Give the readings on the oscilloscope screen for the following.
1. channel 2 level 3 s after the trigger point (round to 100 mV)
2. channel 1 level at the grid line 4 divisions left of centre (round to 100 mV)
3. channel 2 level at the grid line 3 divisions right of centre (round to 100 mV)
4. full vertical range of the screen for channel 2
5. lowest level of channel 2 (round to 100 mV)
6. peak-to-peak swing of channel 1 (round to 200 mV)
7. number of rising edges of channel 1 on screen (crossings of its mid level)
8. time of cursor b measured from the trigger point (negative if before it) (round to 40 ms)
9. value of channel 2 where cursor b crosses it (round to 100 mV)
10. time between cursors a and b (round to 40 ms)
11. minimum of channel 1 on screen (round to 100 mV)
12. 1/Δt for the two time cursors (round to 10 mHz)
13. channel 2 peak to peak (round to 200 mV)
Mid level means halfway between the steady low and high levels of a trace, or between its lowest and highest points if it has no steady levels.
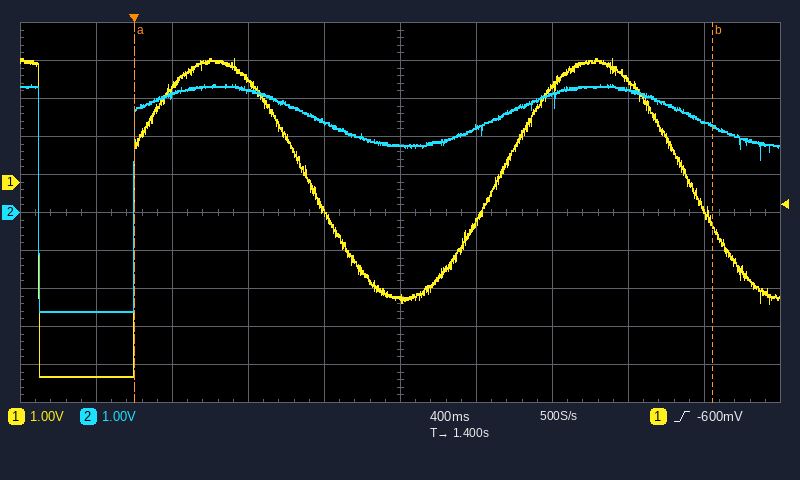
2.4 V
-5.1 V
3.2 V
10 V
-2.6 V
8.4 V
2
+3.04 s
2.3 V
3.04 s
-5.1 V
330 mHz
6.0 V
